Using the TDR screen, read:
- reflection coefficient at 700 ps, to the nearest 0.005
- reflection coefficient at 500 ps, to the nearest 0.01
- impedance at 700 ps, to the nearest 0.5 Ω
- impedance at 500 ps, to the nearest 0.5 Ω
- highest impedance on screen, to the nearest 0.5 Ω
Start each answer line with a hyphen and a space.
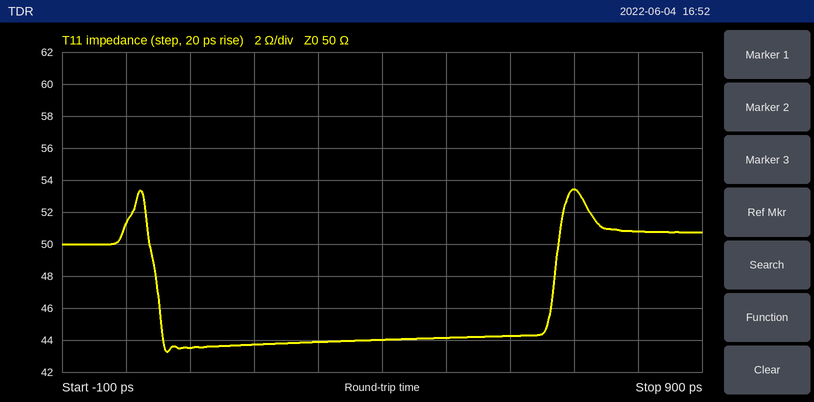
- +0.035
- -0.06
- 53.5 Ω
- 44.0 Ω
- 53.5 Ω
